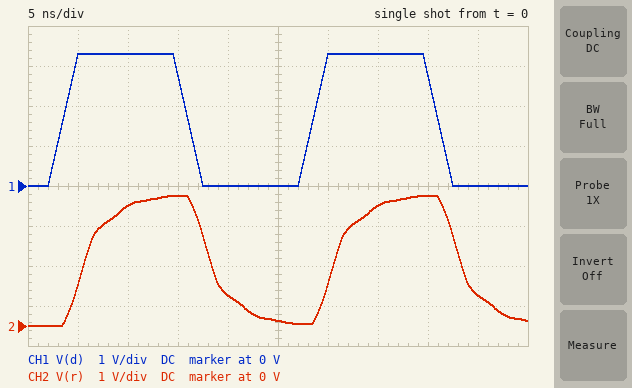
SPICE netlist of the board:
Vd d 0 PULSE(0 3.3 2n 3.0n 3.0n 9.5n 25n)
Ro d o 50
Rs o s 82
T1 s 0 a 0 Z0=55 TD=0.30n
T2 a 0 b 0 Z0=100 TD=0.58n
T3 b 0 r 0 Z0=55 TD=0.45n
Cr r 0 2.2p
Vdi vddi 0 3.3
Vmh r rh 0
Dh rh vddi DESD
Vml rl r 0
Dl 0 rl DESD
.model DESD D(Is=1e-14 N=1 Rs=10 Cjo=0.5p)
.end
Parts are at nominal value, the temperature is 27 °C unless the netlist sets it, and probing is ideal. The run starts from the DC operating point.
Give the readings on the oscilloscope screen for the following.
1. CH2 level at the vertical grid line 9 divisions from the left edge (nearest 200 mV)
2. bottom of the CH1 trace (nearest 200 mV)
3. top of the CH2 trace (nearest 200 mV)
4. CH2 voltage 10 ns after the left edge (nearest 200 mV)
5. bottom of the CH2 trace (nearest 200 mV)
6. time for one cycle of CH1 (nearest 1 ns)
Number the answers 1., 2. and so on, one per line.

1. 800 mV
2. 0 V
3. 3.2 V
4. 3.0 V
5. 0 V
6. 25 ns
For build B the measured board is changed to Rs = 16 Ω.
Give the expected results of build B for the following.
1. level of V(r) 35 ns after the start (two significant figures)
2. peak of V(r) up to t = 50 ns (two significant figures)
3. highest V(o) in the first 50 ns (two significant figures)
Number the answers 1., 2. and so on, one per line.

1. 3.3 V
2. 3.5 V
3. 3.4 V
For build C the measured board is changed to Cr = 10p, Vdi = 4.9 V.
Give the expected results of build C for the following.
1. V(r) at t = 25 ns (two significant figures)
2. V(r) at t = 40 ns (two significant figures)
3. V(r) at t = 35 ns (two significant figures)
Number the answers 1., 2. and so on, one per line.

1. 280 mV
2. 3.2 V
3. 2.7 V
